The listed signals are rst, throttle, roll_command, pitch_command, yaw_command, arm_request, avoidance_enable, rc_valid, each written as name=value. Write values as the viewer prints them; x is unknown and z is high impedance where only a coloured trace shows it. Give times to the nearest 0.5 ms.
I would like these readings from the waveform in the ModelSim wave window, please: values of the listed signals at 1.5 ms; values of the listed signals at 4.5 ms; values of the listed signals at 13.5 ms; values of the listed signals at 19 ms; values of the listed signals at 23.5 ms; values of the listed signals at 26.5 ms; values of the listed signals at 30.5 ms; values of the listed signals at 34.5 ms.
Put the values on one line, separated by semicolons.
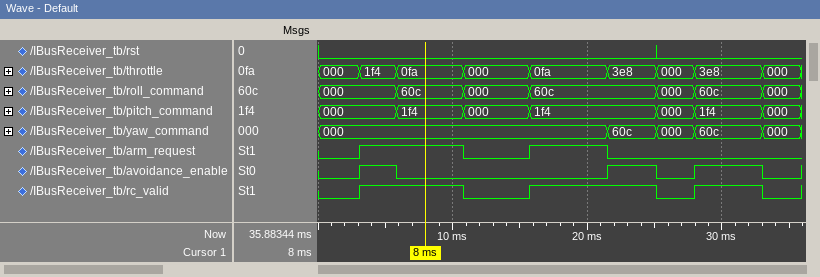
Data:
rst=0, throttle=000, roll_command=000, pitch_command=000, yaw_command=000, arm_request=0, avoidance_enable=0, rc_valid=0; rst=0, throttle=1f4, roll_command=000, pitch_command=000, yaw_command=000, arm_request=1, avoidance_enable=1, rc_valid=1; rst=0, throttle=000, roll_command=000, pitch_command=000, yaw_command=000, arm_request=0, avoidance_enable=0, rc_valid=0; rst=0, throttle=0fa, roll_command=60c, pitch_command=1f4, yaw_command=000, arm_request=1, avoidance_enable=0, rc_valid=1; rst=0, throttle=3e8, roll_command=60c, pitch_command=1f4, yaw_command=60c, arm_request=0, avoidance_enable=1, rc_valid=1; rst=0, throttle=000, roll_command=000, pitch_command=000, yaw_command=000, arm_request=0, avoidance_enable=0, rc_valid=0; rst=0, throttle=3e8, roll_command=60c, pitch_command=1f4, yaw_command=60c, arm_request=0, avoidance_enable=1, rc_valid=1; rst=0, throttle=000, roll_command=000, pitch_command=000, yaw_command=000, arm_request=0, avoidance_enable=0, rc_valid=0
